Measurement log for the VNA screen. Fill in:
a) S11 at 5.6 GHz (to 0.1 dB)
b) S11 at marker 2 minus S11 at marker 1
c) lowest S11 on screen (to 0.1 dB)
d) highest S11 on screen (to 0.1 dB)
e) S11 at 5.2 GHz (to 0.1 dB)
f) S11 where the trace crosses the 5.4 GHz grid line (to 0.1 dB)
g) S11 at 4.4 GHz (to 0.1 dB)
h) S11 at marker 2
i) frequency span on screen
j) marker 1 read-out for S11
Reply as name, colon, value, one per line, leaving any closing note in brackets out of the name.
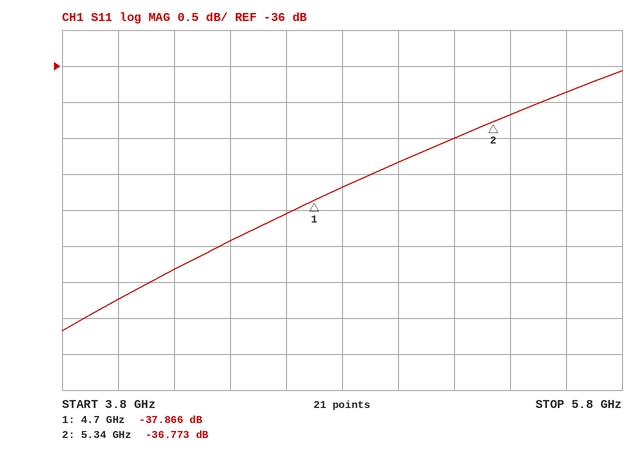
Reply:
S11 at 5.6 GHz: -36.4 dB
S11 at marker 2 minus S11 at marker 1: 1.093 dB
lowest S11 on screen: -39.7 dB
highest S11 on screen: -36.1 dB
S11 at 5.2 GHz: -37.0 dB
S11 where the trace crosses the 5.4 GHz grid line: -36.7 dB
S11 at 4.4 GHz: -38.4 dB
S11 at marker 2: -36.773 dB
frequency span on screen: 2 GHz
marker 1 read-out for S11: -37.866 dB
